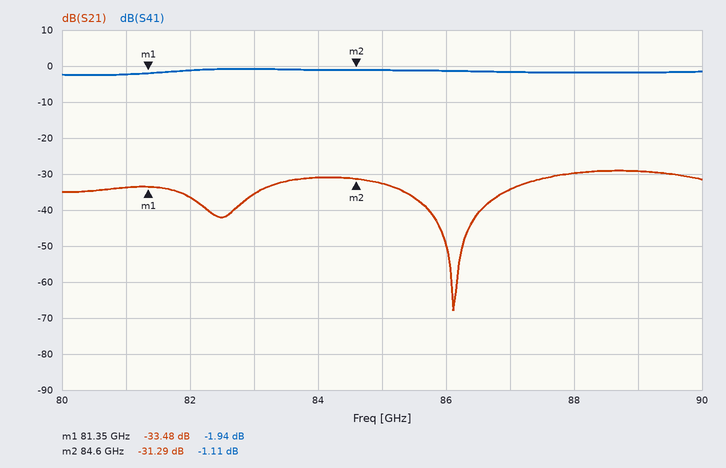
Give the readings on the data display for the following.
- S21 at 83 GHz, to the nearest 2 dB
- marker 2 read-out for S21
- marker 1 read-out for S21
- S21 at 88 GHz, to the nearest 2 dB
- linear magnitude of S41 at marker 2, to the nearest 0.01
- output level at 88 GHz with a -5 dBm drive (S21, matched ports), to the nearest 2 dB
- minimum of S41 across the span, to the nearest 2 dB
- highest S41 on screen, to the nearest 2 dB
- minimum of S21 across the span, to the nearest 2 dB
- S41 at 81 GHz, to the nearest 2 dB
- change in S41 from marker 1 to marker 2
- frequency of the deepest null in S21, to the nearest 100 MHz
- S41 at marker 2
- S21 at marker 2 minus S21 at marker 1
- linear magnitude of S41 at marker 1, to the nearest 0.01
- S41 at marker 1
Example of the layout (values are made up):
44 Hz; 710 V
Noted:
-36 dB; -31.29 dB; -33.48 dB; -30 dB; 0.88; -34 dBm; -2 dB; 0 dB; -68 dB; -2 dB; 0.83 dB; 86.1 GHz; -1.11 dB; 2.19 dB; 0.80; -1.94 dB
